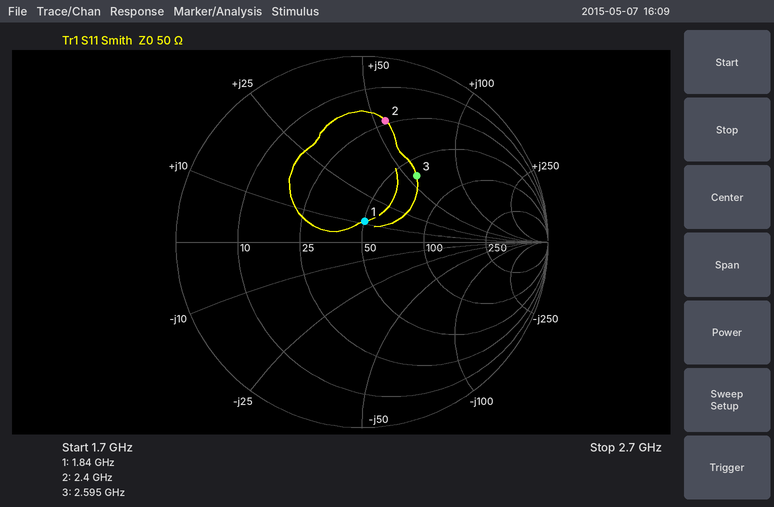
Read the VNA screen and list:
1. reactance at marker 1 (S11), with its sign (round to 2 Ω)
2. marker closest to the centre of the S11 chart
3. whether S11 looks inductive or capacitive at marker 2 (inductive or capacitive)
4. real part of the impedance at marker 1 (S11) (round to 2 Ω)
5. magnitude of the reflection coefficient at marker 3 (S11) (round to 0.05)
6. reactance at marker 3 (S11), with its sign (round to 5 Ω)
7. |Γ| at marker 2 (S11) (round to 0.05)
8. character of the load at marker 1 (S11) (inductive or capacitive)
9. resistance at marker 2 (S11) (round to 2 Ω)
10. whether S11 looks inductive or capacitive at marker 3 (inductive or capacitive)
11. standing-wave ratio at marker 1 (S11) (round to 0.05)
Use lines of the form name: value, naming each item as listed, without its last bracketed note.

reactance at marker 1 (S11), with its sign: +12 Ω
marker closest to the centre of the S11 chart: marker 1
whether S11 looks inductive or capacitive at marker 2: inductive
real part of the impedance at marker 1 (S11): 50 Ω
magnitude of the reflection coefficient at marker 3 (S11): 0.45
reactance at marker 3 (S11), with its sign: +55 Ω
|Γ| at marker 2 (S11): 0.65
character of the load at marker 1 (S11): inductive
resistance at marker 2 (S11): 24 Ω
whether S11 looks inductive or capacitive at marker 3: inductive
standing-wave ratio at marker 1 (S11): 1.25
